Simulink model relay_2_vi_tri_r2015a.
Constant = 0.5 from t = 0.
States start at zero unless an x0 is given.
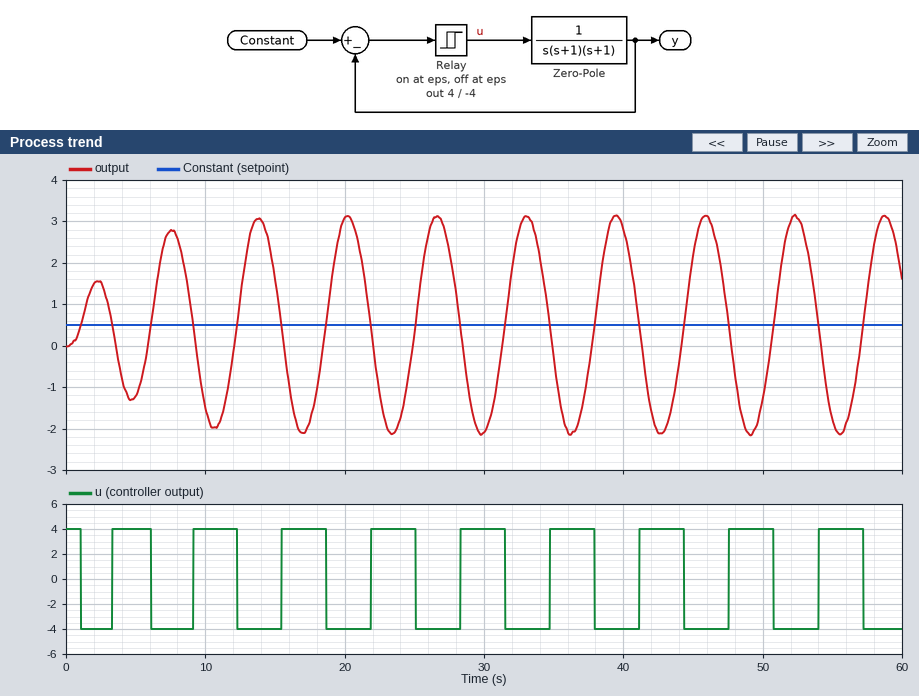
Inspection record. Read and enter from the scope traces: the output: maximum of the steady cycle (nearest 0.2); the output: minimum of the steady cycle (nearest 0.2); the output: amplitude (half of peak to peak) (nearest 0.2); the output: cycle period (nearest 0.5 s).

3.2
-2.2
2.6
6.5 s
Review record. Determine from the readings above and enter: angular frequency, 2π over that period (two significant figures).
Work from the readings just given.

0.97 rad/s
